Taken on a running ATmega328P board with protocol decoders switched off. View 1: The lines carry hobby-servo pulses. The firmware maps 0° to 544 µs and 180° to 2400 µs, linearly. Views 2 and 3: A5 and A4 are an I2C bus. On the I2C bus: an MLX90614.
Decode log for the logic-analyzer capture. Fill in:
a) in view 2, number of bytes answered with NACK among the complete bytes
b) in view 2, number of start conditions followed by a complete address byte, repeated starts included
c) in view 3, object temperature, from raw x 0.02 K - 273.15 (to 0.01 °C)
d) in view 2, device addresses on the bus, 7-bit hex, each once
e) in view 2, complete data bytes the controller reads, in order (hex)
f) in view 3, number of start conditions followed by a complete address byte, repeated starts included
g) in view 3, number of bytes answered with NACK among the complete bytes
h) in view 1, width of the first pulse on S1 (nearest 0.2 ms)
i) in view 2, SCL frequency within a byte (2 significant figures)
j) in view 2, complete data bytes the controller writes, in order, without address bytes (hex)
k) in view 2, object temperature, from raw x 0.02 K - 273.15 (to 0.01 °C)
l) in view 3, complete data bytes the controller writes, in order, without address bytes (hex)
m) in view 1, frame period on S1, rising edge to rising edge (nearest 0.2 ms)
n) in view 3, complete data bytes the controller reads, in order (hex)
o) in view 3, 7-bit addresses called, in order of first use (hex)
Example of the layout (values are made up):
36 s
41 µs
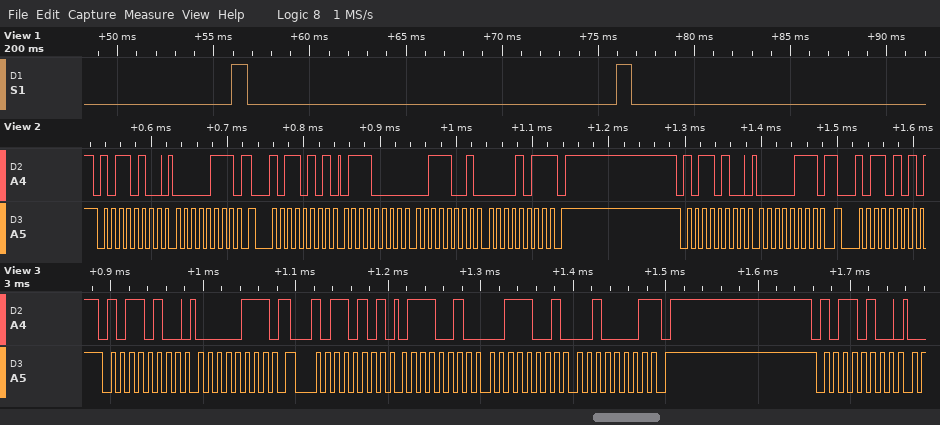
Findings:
1
4
20.97 °C
0x5A
70 39 0B
3
1
0.8 ms
100 kHz
07 07
20.93 °C
07
20.0 ms
72 39 21
0x5A
